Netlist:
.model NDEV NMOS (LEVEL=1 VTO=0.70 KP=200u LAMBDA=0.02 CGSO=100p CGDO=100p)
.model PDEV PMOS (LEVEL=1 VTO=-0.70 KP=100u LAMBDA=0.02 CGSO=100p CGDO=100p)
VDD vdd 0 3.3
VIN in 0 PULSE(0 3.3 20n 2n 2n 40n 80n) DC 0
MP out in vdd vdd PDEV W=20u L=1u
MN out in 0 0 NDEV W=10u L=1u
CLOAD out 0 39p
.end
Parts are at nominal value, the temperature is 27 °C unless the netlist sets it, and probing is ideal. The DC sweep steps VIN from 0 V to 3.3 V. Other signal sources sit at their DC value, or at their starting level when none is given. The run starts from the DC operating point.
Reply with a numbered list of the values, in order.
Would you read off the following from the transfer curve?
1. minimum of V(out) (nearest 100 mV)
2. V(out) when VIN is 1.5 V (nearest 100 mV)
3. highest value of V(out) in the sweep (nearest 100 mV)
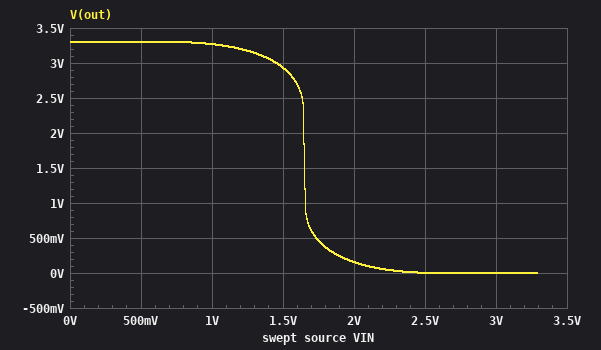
1. 0 V
2. 2.9 V
3. 3.3 V
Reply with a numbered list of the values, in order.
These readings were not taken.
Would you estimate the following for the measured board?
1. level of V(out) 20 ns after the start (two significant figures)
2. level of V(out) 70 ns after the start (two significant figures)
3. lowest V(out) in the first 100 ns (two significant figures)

1. 3.3 V
2. 1.2 V
3. 34 mV
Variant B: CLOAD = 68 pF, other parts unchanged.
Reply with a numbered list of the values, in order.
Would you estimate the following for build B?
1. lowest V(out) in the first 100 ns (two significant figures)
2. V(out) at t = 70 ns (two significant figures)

1. 330 mV
2. 1.0 V
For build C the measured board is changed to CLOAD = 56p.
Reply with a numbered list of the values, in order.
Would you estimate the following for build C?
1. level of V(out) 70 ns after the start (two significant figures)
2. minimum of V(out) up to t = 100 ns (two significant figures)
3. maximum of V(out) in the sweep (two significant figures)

1. 1.0 V
2. 170 mV
3. 3.3 V
